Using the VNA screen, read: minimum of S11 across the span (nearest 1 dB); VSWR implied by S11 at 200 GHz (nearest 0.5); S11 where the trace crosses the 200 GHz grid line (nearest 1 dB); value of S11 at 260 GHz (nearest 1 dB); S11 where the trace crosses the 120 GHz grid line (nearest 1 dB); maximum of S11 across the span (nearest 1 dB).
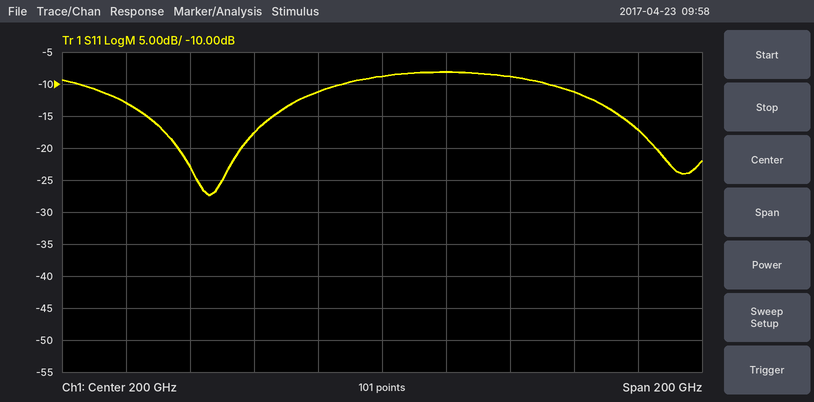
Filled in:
-27 dB
2.0
-9 dB
-11 dB
-13 dB
-8 dB
